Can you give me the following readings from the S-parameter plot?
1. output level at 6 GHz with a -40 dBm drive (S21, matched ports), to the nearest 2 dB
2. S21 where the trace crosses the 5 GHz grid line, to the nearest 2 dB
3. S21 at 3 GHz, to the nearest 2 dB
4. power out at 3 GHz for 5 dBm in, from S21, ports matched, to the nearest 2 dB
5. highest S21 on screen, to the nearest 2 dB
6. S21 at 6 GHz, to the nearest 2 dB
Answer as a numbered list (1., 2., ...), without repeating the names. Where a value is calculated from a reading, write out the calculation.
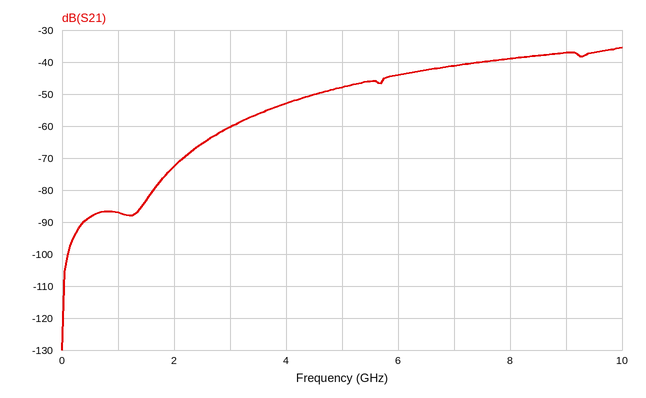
1. -40 dBm + (-44 dB) = -84 dBm
2. -48 dB
3. -60 dB
4. 5 dBm + (-60 dB) = -56 dBm
5. -36 dB
6. -44 dB
